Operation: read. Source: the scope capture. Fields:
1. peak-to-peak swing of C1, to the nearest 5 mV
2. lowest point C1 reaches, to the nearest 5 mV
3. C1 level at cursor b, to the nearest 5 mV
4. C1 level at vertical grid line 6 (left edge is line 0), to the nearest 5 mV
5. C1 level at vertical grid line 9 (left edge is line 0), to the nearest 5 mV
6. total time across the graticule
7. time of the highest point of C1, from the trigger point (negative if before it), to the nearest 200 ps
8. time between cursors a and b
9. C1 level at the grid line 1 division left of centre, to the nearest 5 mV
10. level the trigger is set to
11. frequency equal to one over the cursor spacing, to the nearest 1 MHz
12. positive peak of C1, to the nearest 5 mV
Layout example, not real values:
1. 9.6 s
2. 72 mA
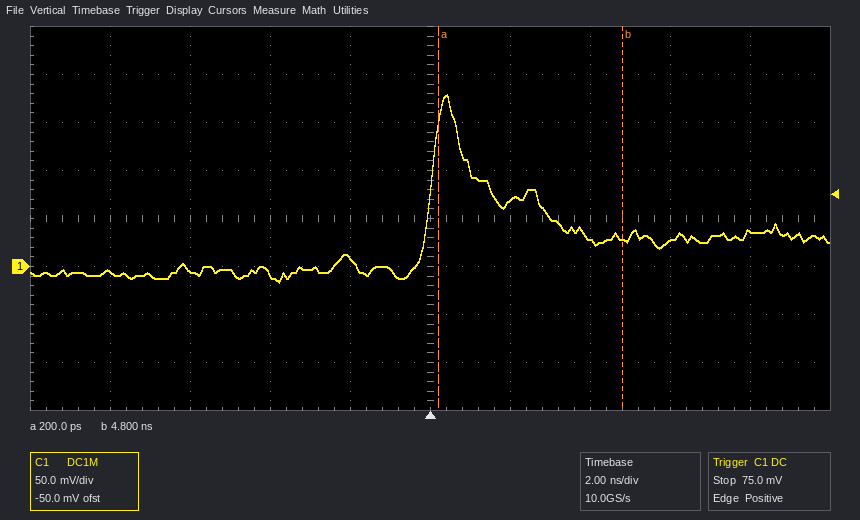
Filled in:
1. 195 mV
2. -15 mV
3. 30 mV
4. 70 mV
5. 35 mV
6. 20 ns
7. +400 ps
8. 4.6 ns
9. 10 mV
10. 75.0 mV
11. 217 MHz
12. 180 mV
